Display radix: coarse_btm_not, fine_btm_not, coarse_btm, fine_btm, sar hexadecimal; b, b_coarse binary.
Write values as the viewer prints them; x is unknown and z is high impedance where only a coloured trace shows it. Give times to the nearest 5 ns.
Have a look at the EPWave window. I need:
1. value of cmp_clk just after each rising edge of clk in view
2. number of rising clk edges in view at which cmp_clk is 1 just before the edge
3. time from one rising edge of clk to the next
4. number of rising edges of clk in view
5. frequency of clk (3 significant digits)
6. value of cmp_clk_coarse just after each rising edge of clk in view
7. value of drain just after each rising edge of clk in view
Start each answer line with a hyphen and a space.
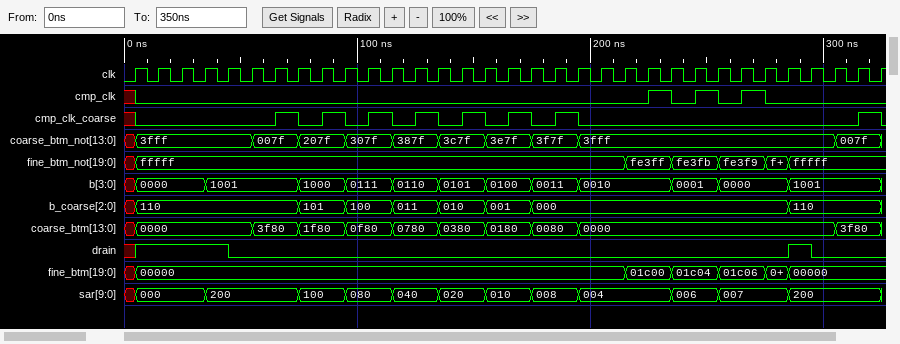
- 0 0 0 0 0 0 0 0 0 0 0 0 0 0 0 0 0 0 0 0 0 0 1 0 1 0 1 0 0 0 0 0 0
- 3
- 10 ns
- 33
- 100 MHz
- 0 0 0 0 0 0 1 0 1 0 1 0 1 0 1 0 1 0 1 0 0 0 0 0 0 0 0 0 0 0 0 1 0
- 1 1 1 1 0 0 0 0 0 0 0 0 0 0 0 0 0 0 0 0 0 0 0 0 0 0 0 0 1 0 0 0 0
